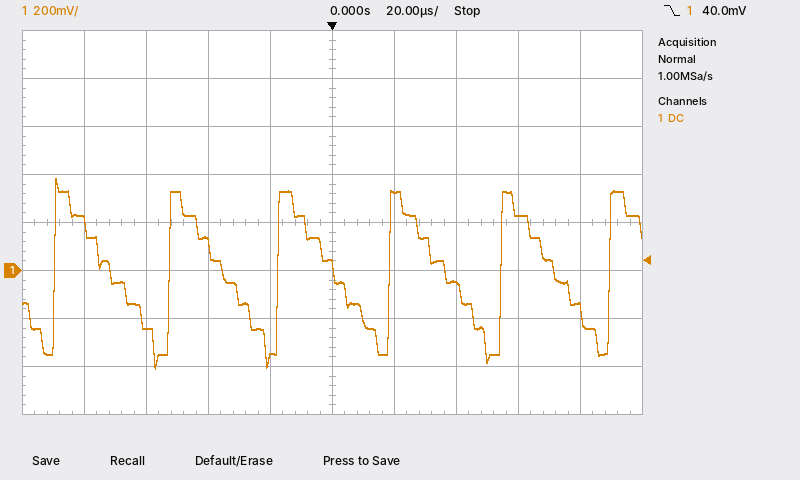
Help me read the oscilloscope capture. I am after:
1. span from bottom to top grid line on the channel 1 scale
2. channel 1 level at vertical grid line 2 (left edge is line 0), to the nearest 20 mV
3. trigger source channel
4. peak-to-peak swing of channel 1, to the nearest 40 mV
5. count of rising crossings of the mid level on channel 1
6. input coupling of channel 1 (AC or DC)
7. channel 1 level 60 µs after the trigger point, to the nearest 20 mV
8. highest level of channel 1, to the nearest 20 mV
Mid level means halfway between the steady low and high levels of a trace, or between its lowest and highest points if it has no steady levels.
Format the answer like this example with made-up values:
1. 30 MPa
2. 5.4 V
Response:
1. 1.6 V
2. -240 mV
3. channel 1
4. 800 mV
5. 6
6. DC
7. 220 mV
8. 380 mV
